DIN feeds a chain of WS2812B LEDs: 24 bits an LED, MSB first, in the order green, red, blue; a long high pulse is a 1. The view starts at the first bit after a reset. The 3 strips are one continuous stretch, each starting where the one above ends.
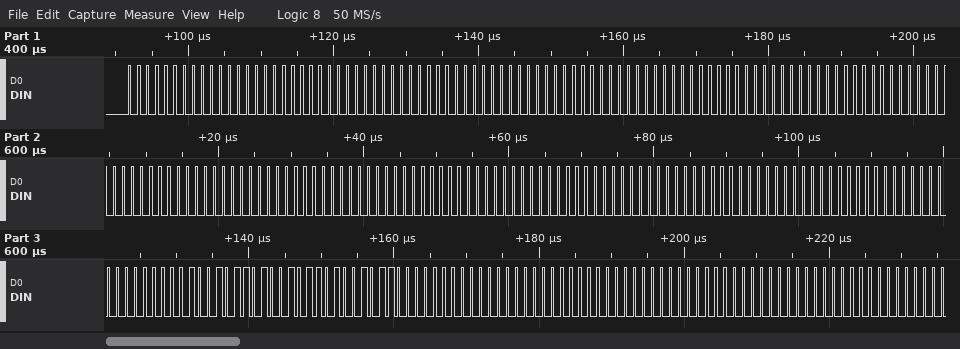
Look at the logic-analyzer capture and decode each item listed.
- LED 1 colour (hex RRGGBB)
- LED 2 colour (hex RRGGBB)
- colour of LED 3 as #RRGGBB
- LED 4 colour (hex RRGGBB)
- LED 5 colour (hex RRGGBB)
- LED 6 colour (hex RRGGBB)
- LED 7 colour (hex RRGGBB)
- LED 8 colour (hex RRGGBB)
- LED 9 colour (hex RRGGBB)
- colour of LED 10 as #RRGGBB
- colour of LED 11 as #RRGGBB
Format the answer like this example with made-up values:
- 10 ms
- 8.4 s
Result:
- #000000
- #000000
- #000000
- #000000
- #000000
- #000000
- #000000
- #000000
- #969696
- #000000
- #000000
